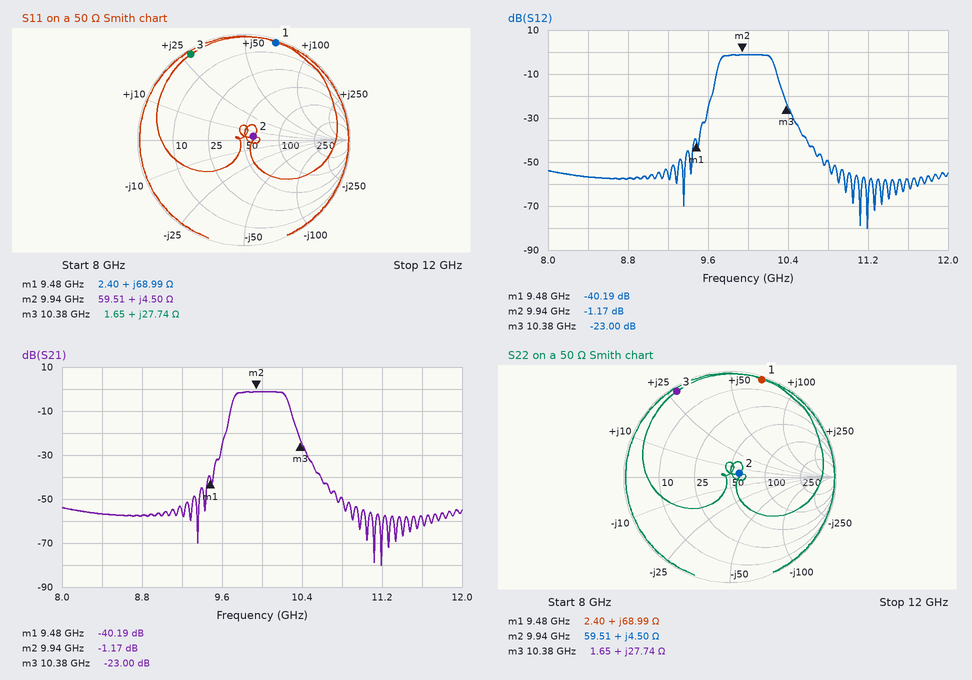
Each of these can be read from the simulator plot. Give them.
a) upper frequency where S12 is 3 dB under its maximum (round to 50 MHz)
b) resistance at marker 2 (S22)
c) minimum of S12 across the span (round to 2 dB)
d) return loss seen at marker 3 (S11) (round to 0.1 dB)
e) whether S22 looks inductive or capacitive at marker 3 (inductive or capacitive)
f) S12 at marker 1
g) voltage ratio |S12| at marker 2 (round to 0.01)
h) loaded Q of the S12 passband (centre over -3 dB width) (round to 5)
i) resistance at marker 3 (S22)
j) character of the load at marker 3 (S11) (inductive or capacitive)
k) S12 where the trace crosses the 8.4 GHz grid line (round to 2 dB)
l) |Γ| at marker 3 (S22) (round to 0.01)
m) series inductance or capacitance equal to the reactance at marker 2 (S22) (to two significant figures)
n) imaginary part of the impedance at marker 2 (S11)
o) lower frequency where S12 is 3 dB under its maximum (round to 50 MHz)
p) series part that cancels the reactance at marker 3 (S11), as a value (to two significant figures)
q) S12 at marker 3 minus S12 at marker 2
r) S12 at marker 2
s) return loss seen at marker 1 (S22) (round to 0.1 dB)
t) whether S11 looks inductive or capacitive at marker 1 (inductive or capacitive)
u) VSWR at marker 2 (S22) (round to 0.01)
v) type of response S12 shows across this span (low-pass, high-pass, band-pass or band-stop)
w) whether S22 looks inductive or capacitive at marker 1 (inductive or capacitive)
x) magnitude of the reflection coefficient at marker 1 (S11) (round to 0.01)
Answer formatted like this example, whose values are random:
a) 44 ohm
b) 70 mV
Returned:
a) 10.25 GHz
b) 59.51 Ω
c) -80 dB
d) 0.4 dB
e) inductive
f) -40.19 dB
g) 0.87
h) 20
i) 1.65 Ω
j) inductive
k) -56 dB
l) 0.95
m) 72 pH
n) +4.50 Ω
o) 9.70 GHz
p) 550 fF
q) -21.83 dB
r) -1.17 dB
s) 0.3 dB
t) inductive
u) 1.21
v) band-pass
w) inductive
x) 0.97
